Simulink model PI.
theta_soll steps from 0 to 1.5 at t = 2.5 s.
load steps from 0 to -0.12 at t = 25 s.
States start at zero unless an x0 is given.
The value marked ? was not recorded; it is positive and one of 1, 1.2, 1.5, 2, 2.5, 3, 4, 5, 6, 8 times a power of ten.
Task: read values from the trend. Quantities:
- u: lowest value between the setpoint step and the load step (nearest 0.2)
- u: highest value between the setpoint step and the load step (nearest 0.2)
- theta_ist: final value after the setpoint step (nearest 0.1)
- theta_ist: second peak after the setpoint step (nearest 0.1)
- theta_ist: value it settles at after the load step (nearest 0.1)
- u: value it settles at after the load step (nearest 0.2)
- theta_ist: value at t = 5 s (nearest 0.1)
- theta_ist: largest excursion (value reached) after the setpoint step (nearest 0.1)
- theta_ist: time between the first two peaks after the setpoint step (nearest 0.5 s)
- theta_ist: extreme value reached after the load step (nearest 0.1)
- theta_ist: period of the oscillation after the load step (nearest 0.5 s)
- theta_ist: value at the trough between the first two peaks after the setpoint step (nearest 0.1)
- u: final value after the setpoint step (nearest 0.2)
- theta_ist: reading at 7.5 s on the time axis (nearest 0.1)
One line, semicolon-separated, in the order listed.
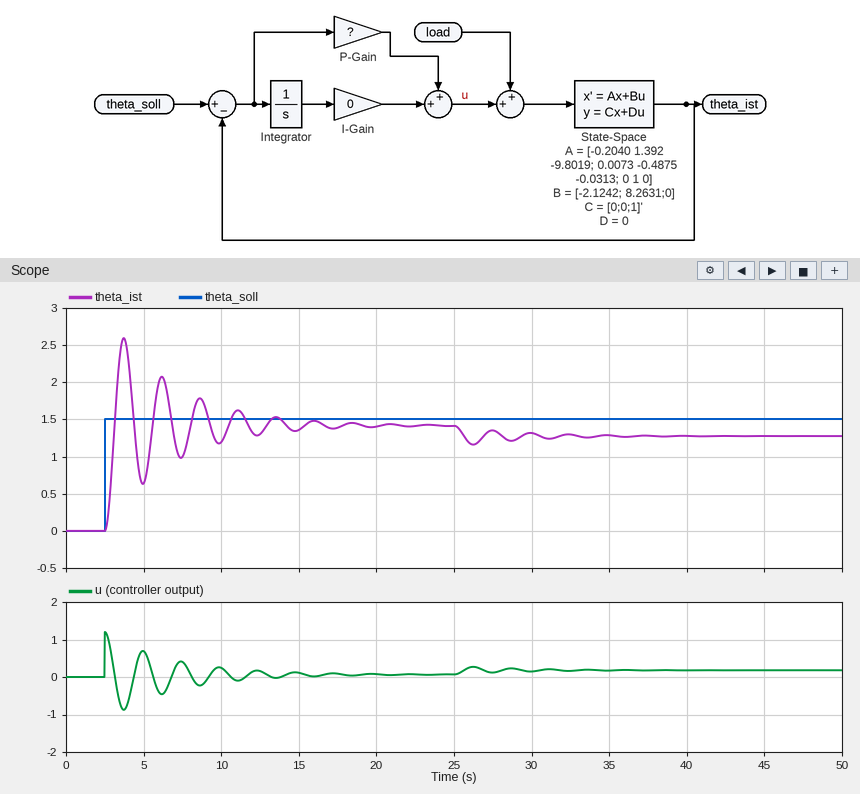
-0.8; 1.2; 1.4; 2.1; 1.3; 0.2; 0.6; 2.6; 2.5 s; 1.2; 2.5 s; 0.6; 0.0; 1.0
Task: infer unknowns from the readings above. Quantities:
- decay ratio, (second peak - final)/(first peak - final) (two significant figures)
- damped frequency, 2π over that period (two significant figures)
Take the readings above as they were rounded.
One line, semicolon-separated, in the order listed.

0.58; 2.5 rad/s
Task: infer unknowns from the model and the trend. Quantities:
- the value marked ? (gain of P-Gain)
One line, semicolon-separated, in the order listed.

0.8
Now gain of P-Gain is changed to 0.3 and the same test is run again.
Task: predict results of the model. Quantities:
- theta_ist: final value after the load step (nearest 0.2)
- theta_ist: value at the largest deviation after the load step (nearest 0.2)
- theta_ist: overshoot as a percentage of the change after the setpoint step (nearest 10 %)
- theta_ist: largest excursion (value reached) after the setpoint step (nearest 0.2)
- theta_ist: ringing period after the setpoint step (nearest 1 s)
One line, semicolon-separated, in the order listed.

1.0; 0.6; 80 %; 2.4; 4 s
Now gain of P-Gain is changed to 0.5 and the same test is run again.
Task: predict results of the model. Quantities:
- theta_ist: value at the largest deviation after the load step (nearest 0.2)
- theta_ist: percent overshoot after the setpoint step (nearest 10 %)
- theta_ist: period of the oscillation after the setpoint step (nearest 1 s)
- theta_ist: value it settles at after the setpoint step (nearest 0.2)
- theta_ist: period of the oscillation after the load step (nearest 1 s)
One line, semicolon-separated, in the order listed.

1.0; 80 %; 3 s; 1.4; 3 s
